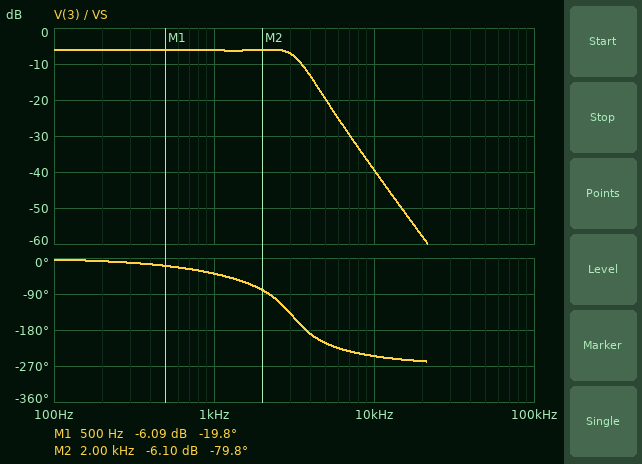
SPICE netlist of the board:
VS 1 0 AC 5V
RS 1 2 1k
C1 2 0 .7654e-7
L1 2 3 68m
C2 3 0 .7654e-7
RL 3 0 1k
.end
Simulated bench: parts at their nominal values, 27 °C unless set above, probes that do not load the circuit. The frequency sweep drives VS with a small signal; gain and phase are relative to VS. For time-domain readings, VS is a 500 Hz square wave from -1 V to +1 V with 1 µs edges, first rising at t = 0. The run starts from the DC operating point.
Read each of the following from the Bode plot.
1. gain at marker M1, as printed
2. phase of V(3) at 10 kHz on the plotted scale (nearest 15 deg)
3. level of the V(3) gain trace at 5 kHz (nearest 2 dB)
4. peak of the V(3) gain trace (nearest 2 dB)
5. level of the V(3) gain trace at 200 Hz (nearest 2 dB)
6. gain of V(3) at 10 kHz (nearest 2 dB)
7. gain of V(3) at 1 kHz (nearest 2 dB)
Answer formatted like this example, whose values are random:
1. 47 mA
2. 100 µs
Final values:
1. -6.09 dB
2. -240 deg
3. -20 dB
4. -6 dB
5. -6 dB
6. -40 dB
7. -6 dB
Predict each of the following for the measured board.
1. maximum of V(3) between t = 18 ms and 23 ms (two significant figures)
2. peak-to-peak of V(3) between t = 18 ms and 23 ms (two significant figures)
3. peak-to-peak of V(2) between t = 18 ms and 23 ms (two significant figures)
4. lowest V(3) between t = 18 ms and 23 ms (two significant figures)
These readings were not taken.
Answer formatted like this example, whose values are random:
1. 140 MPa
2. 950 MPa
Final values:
1. 600 mV
2. 1.2 V
3. 1.2 V
4. -600 mV
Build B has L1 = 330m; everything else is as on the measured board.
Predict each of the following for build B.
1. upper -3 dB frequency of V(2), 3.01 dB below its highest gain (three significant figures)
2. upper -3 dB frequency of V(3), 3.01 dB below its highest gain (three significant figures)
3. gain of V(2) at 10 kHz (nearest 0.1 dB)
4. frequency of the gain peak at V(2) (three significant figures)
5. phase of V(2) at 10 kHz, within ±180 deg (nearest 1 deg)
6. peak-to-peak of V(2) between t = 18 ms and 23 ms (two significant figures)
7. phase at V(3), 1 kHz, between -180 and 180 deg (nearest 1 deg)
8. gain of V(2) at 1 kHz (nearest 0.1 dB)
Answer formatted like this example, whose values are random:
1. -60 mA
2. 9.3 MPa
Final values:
1. 2.99 kHz
2. 1.15 kHz
3. -13.7 dB
4. 1.41 kHz
5. -78 deg
6. 2.0 V
7. -90 deg
8. -1.8 dB
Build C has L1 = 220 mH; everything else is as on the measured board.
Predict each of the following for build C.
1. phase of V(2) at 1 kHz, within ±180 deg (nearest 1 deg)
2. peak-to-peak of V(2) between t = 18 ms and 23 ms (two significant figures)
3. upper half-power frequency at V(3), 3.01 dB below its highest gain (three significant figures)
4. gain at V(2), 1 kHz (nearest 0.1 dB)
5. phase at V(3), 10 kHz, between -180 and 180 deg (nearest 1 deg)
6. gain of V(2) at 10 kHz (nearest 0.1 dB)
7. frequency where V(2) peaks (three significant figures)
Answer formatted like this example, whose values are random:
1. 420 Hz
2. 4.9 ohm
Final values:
1. 5 deg
2. 1.8 V
3. 1.61 kHz
4. -3.5 dB
5. 114 deg
6. -13.7 dB
7. 1.76 kHz
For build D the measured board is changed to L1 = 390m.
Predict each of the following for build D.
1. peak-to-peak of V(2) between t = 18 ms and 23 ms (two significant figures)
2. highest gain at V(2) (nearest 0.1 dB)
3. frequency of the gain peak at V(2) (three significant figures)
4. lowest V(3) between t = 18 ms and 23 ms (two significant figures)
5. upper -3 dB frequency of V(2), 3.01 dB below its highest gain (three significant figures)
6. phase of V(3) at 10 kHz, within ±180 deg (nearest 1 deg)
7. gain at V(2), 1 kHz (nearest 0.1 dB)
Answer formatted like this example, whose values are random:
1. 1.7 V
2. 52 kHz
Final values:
1. 2.1 V
2. -1.0 dB
3. 1.29 kHz
4. -510 mV
5. 2.88 kHz
6. 114 deg
7. -1.3 dB
